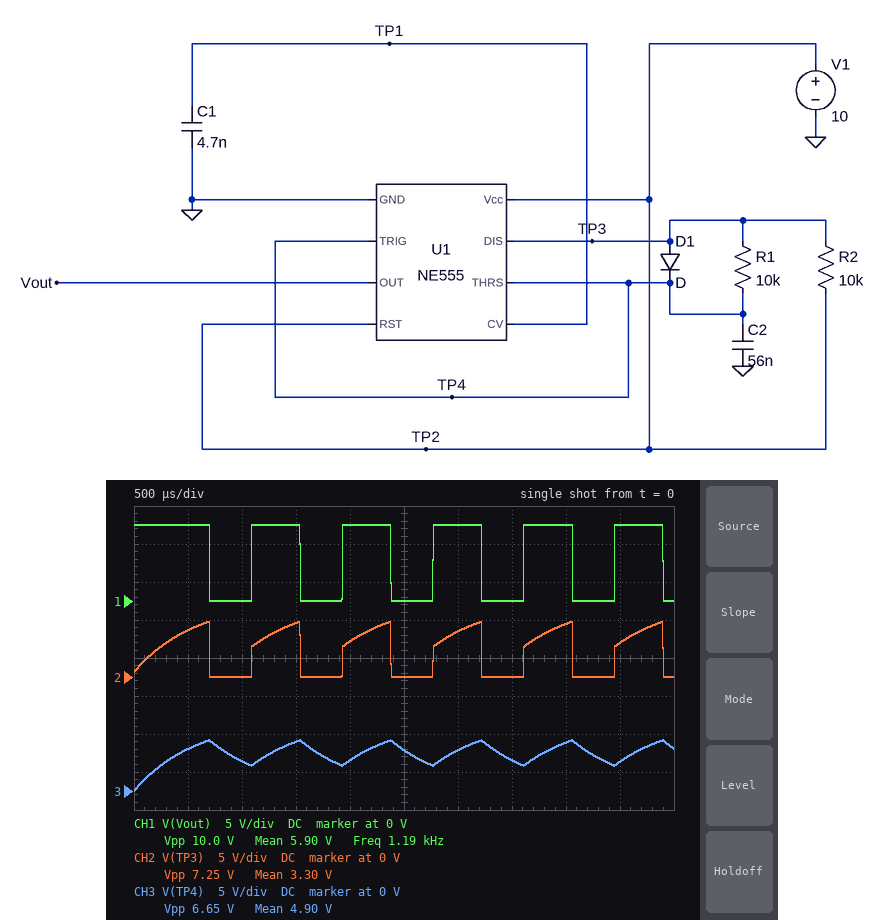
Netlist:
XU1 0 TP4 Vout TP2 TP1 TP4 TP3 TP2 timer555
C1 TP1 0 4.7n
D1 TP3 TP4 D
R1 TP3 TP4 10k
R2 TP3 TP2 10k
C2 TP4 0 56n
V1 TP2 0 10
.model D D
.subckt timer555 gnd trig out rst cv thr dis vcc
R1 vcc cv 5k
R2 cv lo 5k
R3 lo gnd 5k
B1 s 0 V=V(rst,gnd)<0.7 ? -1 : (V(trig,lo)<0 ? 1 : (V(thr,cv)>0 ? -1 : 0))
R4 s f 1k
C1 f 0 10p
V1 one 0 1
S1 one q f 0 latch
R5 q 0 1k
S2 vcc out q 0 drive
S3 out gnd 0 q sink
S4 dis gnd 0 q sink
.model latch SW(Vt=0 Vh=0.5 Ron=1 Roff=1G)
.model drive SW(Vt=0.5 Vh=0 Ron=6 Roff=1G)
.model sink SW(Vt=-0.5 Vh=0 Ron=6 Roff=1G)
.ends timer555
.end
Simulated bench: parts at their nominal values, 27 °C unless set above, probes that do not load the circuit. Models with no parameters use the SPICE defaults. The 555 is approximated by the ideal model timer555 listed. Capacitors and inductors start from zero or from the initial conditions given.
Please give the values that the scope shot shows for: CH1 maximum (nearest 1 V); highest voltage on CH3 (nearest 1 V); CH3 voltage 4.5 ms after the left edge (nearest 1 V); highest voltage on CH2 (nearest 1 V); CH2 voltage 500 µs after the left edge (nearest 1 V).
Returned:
10 V
7 V
4 V
7 V
6 V
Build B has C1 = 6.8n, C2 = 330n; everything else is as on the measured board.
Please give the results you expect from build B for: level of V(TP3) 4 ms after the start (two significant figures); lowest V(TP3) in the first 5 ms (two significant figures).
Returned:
7.2 V
9.0 mV
